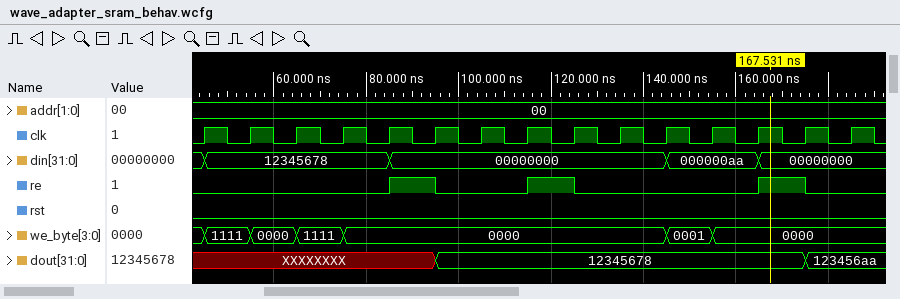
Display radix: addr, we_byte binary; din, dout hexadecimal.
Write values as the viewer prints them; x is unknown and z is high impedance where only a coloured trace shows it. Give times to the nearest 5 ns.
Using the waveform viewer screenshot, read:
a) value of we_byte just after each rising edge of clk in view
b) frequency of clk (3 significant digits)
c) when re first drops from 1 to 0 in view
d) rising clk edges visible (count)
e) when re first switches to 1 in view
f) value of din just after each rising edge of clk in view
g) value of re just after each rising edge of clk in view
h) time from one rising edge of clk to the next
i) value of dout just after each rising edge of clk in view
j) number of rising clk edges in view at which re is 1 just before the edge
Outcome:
1111, 0000, 1111, 0000, 0000, 0000, 0000, 0000, 0000, 0000, 0001, 0000, 0000, 0000, 0000
100 MHz
95 ns
15
85 ns
12345678, 12345678, 12345678, 12345678, 00000000, 00000000, 00000000, 00000000, 00000000, 00000000, 000000aa, 000000aa, 00000000, 00000000, 00000000
0 0 0 0 1 0 0 1 0 0 0 0 1 0 0
10 ns
XXXXXXXX, XXXXXXXX, XXXXXXXX, XXXXXXXX, XXXXXXXX, 12345678, 12345678, 12345678, 12345678, 12345678, 12345678, 12345678, 12345678, 123456aa, 123456aa
3
